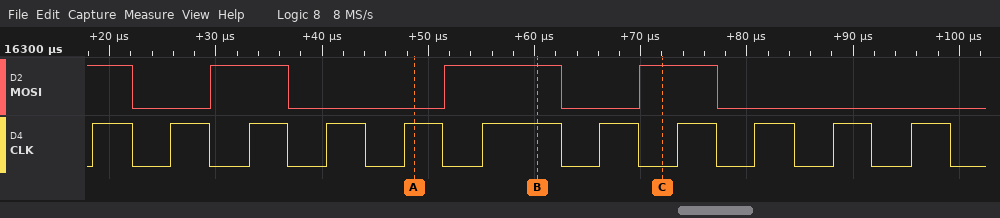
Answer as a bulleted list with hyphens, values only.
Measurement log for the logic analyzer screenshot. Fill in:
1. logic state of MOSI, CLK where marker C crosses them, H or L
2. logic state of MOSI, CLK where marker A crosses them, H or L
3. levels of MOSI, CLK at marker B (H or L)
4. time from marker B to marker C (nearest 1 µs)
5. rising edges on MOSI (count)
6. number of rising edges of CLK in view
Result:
- MOSI=H, CLK=L
- MOSI=L, CLK=H
- MOSI=H, CLK=H
- 12 µs
- 3
- 11
